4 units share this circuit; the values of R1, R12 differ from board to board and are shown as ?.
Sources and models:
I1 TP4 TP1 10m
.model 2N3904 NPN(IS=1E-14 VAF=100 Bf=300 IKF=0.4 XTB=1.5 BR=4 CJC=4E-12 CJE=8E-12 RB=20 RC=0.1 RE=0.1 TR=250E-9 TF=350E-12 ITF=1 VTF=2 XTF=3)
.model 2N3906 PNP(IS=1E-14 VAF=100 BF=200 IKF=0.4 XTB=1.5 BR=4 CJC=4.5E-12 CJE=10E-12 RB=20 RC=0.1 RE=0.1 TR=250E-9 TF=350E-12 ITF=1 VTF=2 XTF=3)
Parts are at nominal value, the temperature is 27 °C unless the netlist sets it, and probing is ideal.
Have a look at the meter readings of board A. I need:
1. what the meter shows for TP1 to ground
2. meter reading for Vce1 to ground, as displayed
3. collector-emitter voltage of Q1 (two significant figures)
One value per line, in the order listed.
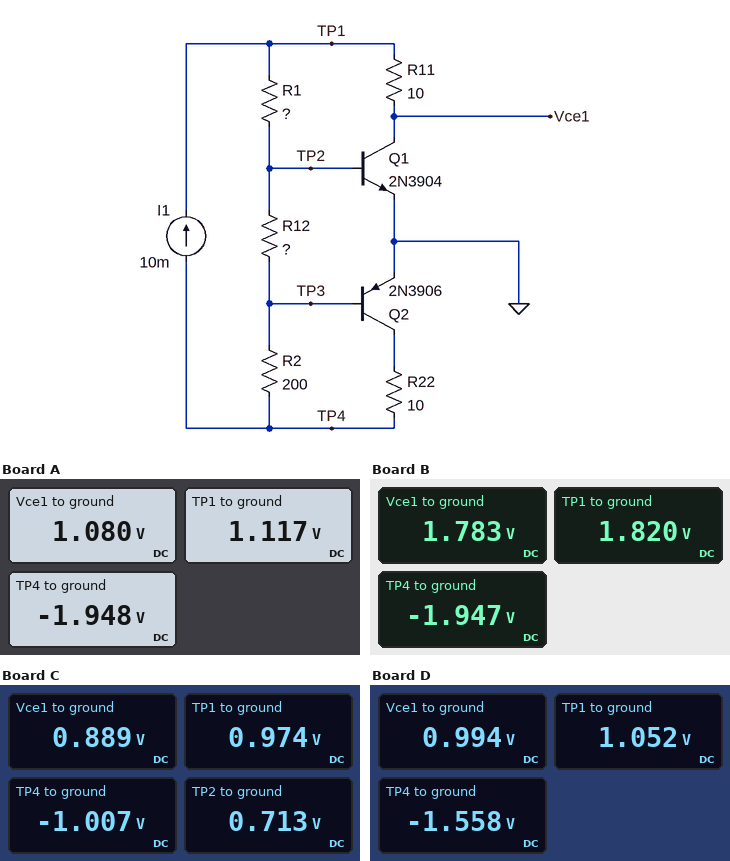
1.117 V
1.080 V
1.1 V
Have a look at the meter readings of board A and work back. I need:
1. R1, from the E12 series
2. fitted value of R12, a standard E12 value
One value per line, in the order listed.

68 Ω
220 Ω
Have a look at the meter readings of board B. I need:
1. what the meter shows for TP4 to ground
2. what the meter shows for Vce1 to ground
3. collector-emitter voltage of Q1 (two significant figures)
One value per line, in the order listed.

-1.947 V
1.783 V
1.8 V
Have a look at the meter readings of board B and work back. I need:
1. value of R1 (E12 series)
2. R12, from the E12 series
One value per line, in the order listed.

180 Ω
220 Ω
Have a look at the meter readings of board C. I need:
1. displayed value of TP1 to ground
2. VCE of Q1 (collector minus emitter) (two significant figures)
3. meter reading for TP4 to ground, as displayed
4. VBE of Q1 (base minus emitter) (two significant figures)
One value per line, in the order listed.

0.974 V
890 mV
-1.007 V
710 mV
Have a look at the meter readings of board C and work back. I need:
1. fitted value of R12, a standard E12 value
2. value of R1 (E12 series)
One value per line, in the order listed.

1 kΩ
180 Ω
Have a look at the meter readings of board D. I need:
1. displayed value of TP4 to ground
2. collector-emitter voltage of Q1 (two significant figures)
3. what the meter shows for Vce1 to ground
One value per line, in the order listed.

-1.558 V
990 mV
0.994 V
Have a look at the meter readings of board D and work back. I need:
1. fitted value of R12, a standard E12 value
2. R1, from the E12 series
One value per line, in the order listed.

330 Ω
82 Ω
